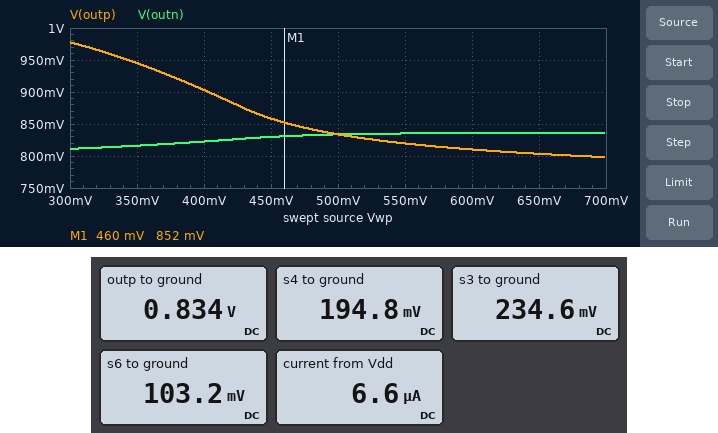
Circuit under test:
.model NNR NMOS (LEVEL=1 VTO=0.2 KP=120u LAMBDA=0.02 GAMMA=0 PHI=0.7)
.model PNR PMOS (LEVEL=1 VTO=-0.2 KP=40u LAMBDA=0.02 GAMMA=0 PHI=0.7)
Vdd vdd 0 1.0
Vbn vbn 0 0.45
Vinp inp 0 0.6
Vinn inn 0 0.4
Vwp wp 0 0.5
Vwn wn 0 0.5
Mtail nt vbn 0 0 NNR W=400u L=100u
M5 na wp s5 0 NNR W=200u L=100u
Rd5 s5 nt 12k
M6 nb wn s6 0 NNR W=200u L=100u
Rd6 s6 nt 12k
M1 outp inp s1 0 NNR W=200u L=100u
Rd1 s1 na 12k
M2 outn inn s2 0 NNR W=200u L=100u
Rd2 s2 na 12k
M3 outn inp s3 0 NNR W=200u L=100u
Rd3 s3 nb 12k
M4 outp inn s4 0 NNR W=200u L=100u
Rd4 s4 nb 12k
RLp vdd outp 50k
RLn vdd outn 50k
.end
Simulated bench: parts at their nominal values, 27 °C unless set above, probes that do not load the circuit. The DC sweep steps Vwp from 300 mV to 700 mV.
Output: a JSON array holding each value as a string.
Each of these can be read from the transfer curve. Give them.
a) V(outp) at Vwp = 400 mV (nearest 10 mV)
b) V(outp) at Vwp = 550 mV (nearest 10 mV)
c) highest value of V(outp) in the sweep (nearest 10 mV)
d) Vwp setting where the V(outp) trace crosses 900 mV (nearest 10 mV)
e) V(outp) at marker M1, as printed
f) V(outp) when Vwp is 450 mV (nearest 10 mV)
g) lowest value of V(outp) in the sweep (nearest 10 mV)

["900 mV", "820 mV", "980 mV", "400 mV", "852 mV", "860 mV", "800 mV"]
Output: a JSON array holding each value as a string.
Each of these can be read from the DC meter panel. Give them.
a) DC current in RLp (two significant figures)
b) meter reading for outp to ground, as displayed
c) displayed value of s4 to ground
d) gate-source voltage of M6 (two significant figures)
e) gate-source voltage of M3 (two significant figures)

["3.3 µA", "0.834 V", "194.8 mV", "400 mV", "370 mV"]
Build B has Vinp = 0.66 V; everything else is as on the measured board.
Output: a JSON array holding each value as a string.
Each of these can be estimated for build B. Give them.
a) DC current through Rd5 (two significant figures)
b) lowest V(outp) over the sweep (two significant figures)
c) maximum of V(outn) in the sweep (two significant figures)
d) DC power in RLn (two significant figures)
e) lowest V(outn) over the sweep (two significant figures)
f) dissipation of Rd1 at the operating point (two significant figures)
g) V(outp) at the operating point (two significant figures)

["3.7 µA", "760 mV", "830 mV", "680 nW", "780 mV", "160 nW", "820 mV"]
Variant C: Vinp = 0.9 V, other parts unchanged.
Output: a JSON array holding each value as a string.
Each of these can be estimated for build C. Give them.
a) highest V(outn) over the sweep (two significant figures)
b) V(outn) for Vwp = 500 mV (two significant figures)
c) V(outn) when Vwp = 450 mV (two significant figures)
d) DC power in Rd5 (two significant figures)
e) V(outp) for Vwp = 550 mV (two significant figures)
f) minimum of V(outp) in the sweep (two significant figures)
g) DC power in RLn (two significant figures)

["860 mV", "810 mV", "790 mV", "180 nW", "750 mV", "620 mV", "740 nW"]
